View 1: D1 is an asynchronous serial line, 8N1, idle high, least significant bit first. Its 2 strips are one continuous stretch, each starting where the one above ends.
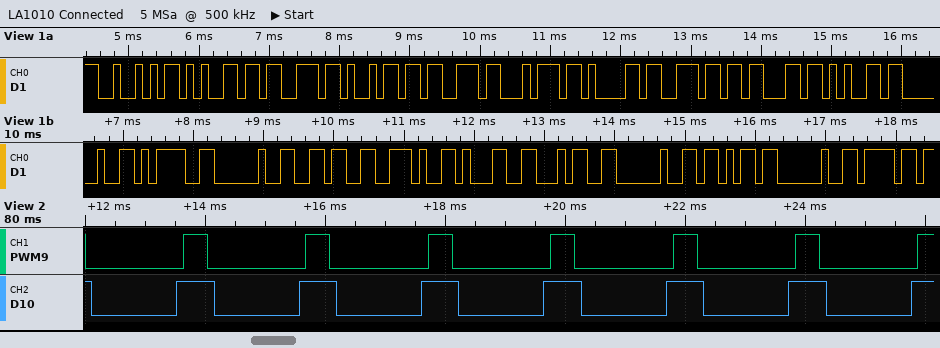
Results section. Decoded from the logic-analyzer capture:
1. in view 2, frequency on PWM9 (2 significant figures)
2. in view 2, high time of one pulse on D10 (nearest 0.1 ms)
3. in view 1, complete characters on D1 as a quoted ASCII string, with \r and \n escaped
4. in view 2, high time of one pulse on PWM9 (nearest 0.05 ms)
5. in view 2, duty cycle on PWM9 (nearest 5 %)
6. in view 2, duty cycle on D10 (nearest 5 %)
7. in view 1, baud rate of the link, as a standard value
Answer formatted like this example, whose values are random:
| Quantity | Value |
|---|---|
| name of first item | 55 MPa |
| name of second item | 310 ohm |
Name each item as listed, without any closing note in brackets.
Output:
| Quantity | Value |
|---|---|
| in view 2, frequency on PWM9 | 490 Hz |
| in view 2, high time of one pulse on D10 | 0.6 ms |
| in view 1, complete characters on D1 as a quoted ASCII string, with \r and \n escaped | "Resistance = 6.14 k o" |
| in view 2, high time of one pulse on PWM9 | 0.40 ms |
| in view 2, duty cycle on PWM9 | 20 % |
| in view 2, duty cycle on D10 | 30 % |
| in view 1, baud rate of the link, as a standard value | 9600 baud |
